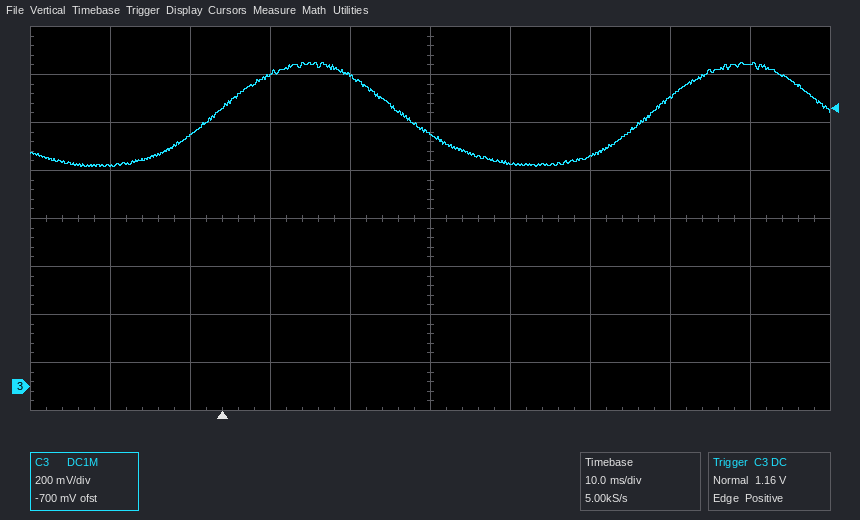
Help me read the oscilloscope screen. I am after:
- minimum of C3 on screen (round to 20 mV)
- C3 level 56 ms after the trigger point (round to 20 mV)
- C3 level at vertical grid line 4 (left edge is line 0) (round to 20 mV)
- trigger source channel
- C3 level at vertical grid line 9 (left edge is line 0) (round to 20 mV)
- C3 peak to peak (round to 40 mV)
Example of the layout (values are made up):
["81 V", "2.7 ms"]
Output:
["920 mV", "1.20 V", "1.30 V", "C3", "1.34 V", "440 mV"]
